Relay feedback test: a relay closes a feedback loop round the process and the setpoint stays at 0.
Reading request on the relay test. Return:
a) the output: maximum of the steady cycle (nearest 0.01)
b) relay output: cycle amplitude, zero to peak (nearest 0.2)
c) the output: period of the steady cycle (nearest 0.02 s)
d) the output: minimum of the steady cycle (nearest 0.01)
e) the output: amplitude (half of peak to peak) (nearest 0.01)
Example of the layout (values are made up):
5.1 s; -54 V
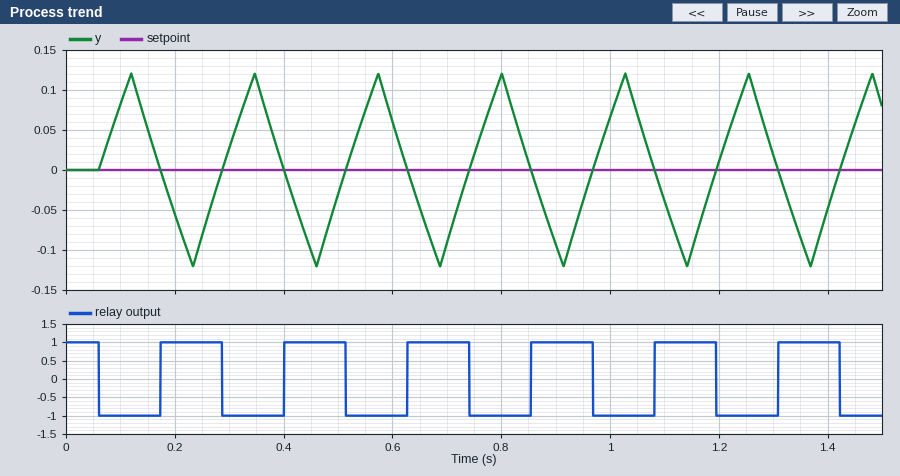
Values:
0.12; 1.0; 0.22 s; -0.12; 0.12
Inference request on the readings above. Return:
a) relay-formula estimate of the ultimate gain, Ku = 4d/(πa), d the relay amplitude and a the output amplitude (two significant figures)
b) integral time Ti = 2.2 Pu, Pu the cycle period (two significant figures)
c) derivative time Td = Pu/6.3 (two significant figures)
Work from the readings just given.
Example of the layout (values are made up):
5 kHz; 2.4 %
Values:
11; 0.48 s; 0.035 s
